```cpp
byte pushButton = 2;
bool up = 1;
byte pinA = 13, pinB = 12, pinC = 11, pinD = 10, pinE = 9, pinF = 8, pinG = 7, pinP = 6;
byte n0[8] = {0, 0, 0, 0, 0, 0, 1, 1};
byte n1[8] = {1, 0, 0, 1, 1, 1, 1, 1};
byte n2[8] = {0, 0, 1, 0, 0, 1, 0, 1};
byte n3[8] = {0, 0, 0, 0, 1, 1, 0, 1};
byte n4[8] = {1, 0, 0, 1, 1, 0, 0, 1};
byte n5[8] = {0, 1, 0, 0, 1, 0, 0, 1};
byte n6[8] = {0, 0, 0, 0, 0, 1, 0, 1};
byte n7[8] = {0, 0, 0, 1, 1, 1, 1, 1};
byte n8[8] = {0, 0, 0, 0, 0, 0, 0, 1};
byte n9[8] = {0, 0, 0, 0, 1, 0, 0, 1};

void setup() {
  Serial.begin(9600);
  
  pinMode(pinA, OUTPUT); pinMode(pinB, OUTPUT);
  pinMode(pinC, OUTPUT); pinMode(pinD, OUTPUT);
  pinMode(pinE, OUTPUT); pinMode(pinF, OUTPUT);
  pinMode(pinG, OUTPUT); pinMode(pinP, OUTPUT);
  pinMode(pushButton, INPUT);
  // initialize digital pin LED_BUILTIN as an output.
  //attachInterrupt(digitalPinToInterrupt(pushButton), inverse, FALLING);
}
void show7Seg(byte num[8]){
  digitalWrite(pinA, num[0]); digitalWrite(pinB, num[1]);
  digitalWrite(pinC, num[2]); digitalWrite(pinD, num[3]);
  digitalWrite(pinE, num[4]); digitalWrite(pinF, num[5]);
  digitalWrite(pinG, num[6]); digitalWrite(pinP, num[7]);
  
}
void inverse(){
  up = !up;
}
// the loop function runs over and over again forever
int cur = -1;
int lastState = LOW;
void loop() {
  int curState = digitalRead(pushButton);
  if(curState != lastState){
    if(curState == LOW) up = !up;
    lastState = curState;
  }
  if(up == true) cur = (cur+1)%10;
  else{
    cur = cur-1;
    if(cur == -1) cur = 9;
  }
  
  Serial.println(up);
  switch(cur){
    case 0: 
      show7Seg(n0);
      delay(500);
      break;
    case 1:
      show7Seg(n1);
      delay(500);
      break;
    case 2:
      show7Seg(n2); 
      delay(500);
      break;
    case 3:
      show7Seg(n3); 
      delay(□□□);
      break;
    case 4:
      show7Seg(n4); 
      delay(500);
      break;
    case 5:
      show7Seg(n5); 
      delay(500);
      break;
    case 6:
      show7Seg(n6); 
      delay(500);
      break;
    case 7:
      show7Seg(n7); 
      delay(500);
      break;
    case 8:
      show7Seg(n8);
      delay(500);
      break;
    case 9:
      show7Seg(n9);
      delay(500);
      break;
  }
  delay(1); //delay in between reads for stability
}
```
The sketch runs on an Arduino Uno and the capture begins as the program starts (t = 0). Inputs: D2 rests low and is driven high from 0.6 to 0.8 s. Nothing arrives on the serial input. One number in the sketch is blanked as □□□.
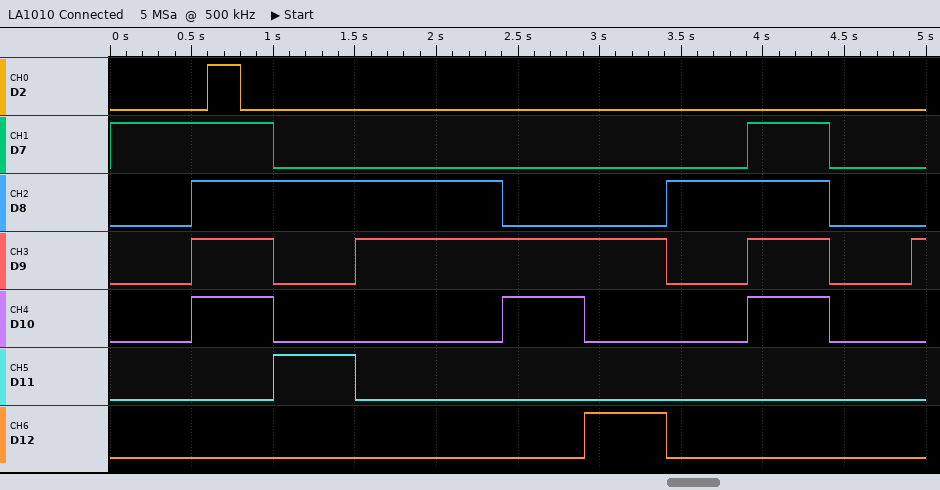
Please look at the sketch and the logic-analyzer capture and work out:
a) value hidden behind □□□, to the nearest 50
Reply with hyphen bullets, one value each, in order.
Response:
- 900
